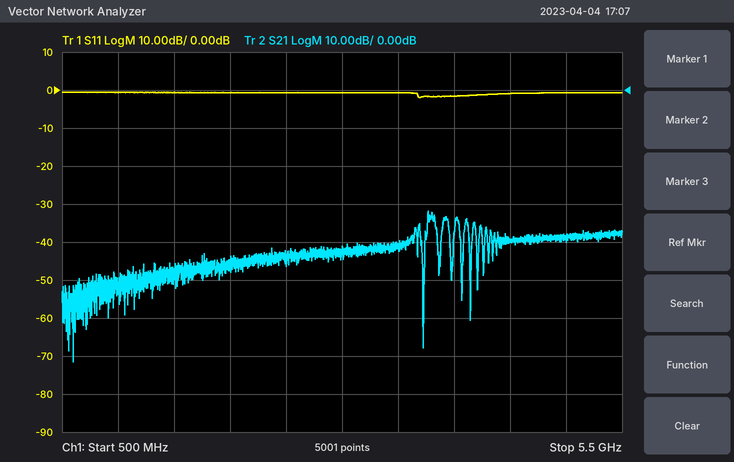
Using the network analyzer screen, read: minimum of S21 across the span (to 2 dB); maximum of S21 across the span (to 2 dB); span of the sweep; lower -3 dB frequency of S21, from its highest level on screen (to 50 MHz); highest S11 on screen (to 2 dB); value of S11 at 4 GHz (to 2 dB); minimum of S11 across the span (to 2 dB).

-72 dB
-32 dB
5 GHz
3.75 GHz
0 dB
-2 dB
-2 dB
